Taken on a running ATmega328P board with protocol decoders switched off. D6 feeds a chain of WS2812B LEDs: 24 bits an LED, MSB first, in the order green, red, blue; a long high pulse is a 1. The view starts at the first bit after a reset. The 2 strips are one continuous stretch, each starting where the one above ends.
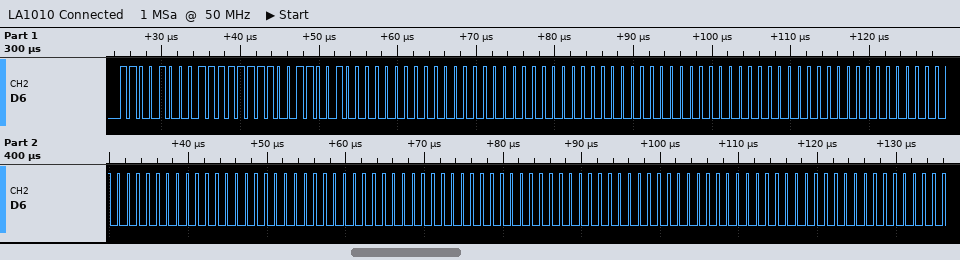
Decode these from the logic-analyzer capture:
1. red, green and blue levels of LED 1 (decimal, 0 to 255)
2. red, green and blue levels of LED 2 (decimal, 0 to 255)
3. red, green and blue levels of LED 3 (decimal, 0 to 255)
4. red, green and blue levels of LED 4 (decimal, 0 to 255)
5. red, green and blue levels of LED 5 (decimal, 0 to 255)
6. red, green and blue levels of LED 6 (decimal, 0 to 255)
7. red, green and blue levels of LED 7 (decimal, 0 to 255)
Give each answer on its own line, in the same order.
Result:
255, 200, 50
0, 0, 0
0, 0, 0
0, 0, 0
0, 0, 0
0, 0, 0
0, 0, 0
